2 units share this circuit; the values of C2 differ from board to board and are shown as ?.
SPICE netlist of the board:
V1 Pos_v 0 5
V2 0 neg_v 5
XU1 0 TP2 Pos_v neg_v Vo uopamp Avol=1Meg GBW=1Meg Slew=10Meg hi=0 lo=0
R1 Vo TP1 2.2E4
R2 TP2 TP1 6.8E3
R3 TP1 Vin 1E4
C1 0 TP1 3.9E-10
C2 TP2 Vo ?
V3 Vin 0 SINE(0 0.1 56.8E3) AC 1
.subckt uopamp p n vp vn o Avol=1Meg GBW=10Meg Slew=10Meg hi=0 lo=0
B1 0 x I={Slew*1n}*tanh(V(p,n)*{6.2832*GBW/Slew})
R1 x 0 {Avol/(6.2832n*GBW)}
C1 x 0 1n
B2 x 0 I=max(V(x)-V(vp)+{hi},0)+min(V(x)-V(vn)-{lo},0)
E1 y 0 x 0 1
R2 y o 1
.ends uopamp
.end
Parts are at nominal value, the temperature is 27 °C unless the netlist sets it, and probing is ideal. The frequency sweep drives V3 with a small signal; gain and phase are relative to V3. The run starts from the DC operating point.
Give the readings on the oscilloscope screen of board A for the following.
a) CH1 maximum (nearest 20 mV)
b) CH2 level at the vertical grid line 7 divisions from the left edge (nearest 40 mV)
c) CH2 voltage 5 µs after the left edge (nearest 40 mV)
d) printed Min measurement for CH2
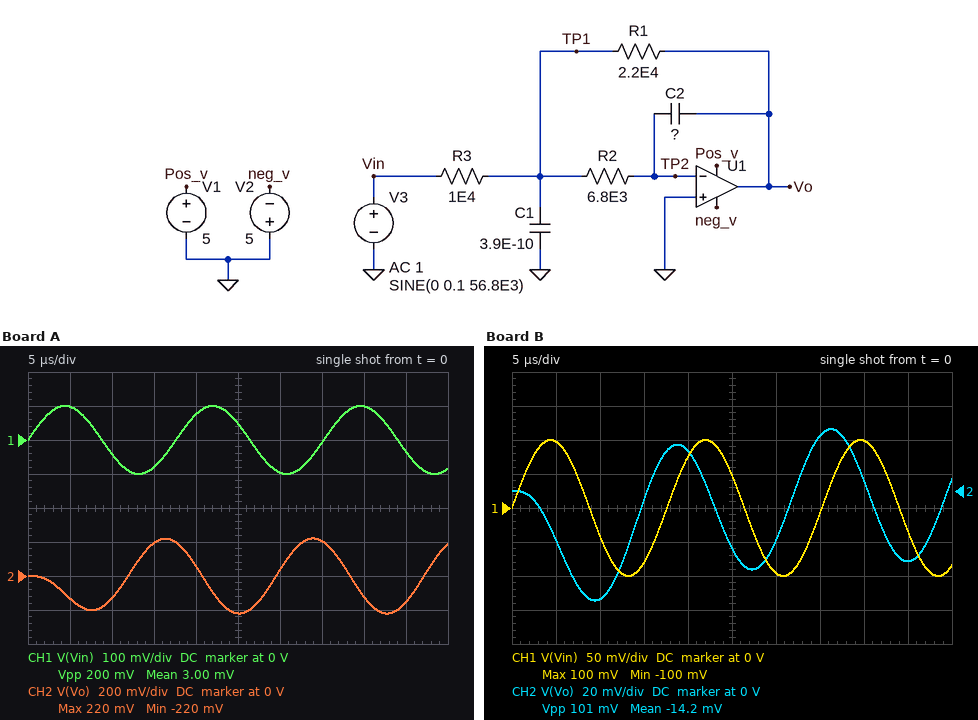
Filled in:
100 mV
200 mV
-120 mV
-220 mV
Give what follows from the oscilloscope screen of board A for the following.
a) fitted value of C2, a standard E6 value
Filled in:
47 pF
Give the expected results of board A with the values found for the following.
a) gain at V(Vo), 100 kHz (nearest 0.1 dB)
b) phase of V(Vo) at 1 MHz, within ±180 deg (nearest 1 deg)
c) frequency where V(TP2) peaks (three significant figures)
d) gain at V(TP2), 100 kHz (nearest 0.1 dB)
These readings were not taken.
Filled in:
2.3 dB
-28 deg
77.8 kHz
-17.7 dB
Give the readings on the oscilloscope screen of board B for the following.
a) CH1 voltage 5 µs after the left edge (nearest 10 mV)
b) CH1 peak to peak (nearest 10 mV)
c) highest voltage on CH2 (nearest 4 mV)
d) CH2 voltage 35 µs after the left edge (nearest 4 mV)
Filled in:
100 mV
200 mV
36 mV
32 mV
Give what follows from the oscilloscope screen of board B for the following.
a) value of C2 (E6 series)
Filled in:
330 pF
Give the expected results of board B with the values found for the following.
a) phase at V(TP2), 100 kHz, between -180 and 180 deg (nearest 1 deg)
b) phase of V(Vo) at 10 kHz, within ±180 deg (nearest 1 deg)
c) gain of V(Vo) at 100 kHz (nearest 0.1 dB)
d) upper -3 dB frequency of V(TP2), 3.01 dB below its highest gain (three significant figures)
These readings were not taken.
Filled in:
-43 deg
134 deg
-14.6 dB
122 kHz
